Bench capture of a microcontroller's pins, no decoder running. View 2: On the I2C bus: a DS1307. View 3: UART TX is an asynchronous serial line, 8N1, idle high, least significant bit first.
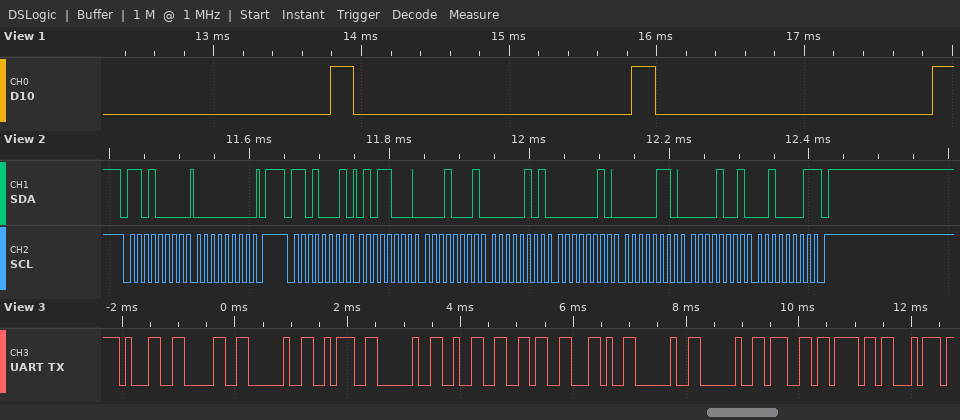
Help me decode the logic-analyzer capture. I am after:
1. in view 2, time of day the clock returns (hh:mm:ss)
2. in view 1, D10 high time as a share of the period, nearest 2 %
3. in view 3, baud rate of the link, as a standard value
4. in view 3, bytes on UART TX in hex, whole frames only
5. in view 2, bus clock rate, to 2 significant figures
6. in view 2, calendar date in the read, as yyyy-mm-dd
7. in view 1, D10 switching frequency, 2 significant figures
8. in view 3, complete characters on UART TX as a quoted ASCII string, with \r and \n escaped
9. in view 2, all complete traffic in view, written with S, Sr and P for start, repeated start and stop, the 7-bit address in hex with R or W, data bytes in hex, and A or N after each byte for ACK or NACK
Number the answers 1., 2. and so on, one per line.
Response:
1. 05:11:58
2. 8 %
3. 9600 baud
4. 0x31 0x30 0x20 0x3A 0x20 0x32 0x36 0x2C 0x20 0x20 0x67 0x6F 0x74
5. 100 kHz
6. 2021-09-06
7. 490 Hz
8. "10 : 26,  got"
9. S 68W A 00 A P S 68R A 58 A 11 A 05 A 02 A 06 A 09 A 21 N P
